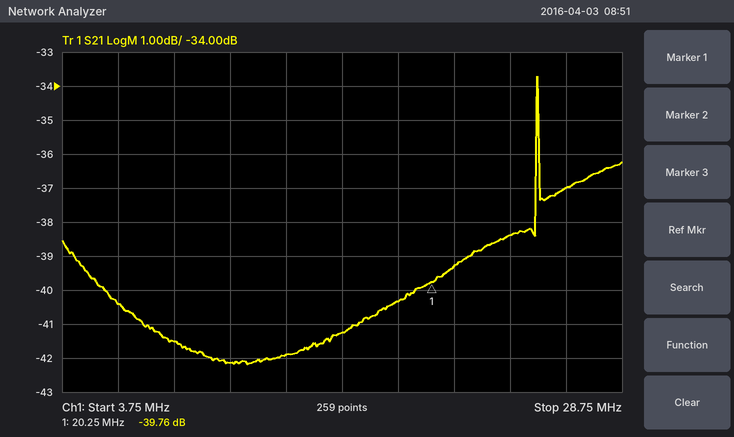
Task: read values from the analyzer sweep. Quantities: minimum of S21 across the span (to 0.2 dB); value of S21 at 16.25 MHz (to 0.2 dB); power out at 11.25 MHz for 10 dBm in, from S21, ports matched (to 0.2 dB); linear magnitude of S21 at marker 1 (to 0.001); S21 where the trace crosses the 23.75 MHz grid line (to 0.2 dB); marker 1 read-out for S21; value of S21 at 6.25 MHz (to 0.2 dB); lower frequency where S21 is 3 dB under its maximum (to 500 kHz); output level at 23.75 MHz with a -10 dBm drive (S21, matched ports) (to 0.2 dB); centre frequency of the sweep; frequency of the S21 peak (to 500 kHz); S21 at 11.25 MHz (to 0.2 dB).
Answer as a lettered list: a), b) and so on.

a) -42.2 dB
b) -41.2 dB
c) -32.2 dBm
d) 0.010
e) -38.4 dB
f) -39.76 dB
g) -40.4 dB
h) 25.0 MHz
i) -48.4 dBm
j) 16.25 MHz
k) 25.0 MHz
l) -42.2 dB
